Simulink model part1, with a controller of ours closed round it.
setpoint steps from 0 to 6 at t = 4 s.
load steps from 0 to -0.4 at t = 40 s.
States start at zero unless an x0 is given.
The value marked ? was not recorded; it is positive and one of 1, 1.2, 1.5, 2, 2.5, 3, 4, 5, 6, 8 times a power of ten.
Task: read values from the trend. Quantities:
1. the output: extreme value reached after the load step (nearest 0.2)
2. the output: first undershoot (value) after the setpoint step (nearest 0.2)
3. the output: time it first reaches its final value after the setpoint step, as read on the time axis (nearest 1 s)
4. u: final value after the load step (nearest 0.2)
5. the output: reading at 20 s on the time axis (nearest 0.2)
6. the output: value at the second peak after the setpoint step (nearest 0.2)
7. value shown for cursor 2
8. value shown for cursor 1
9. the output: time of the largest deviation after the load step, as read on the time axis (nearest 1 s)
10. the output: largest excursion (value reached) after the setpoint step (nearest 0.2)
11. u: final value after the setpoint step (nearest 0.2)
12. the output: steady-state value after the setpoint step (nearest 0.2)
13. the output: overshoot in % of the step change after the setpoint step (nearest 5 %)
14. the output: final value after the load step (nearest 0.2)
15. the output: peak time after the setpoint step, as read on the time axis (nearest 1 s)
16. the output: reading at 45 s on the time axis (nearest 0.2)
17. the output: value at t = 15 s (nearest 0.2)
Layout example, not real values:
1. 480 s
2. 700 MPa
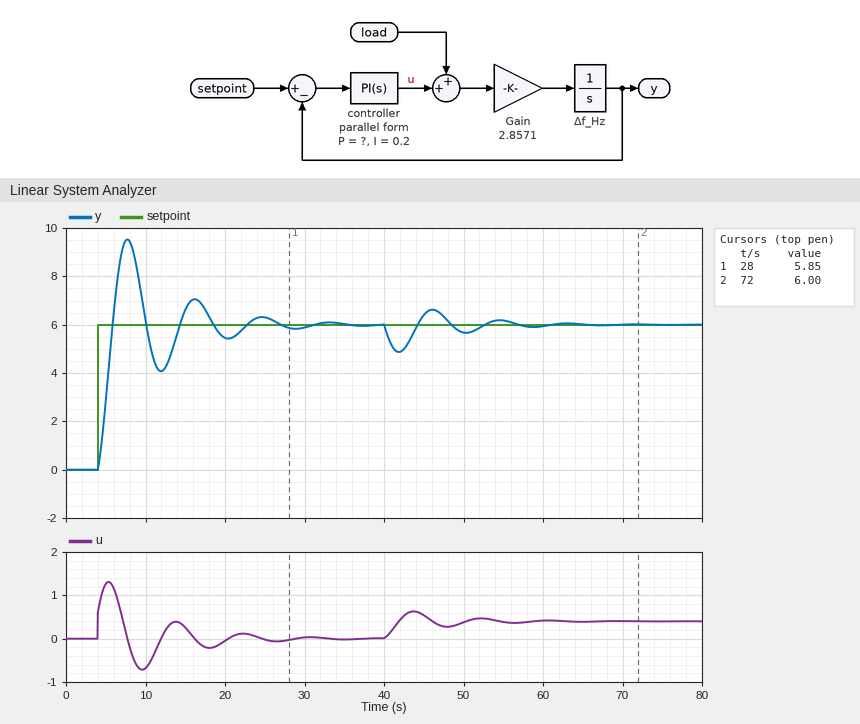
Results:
1. 4.8
2. 4.0
3. 6 s
4. 0.4
5. 5.4
6. 7.0
7. 6.00
8. 5.85
9. 42 s
10. 9.6
11. 0.0
12. 6.0
13. 60 %
14. 6.0
15. 8 s
16. 6.4
17. 6.6
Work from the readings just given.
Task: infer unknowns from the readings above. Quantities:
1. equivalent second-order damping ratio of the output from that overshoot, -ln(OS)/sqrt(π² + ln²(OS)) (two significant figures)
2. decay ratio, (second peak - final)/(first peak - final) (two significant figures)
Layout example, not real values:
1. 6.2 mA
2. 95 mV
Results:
1. 0.16
2. 0.28
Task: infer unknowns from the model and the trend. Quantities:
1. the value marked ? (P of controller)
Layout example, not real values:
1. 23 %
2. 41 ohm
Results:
1. 0.1
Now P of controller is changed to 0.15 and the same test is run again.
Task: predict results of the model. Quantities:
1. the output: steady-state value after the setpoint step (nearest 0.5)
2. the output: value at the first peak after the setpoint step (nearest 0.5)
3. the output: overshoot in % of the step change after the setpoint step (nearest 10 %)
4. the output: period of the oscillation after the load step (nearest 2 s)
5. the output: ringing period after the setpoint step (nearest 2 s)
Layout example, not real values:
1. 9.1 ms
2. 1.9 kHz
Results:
1. 6.0
2. 9.0
3. 50 %
4. 8 s
5. 8 s
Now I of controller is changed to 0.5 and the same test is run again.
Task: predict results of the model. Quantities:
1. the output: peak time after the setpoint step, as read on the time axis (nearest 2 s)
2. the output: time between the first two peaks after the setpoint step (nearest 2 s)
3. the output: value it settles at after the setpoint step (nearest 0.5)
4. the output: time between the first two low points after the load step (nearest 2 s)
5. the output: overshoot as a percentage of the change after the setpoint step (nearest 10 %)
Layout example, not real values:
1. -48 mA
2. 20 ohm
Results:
1. 6 s
2. 6 s
3. 6.0
4. 6 s
5. 70 %
